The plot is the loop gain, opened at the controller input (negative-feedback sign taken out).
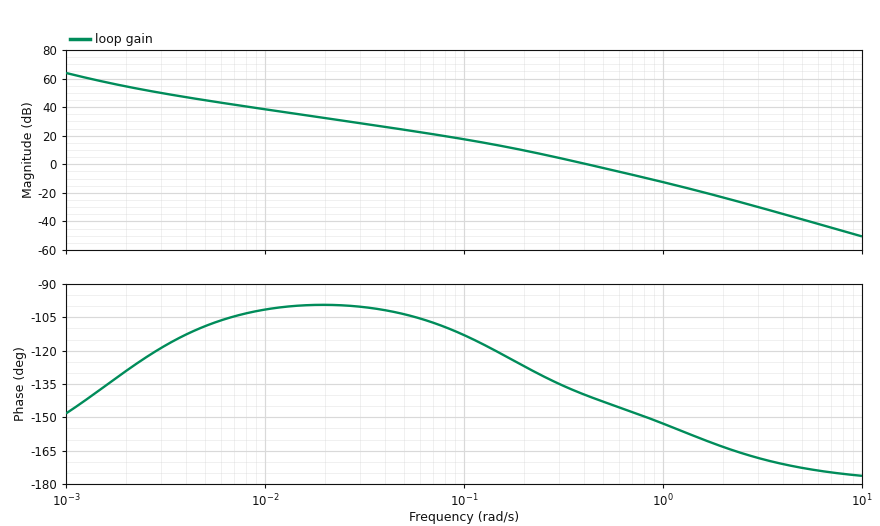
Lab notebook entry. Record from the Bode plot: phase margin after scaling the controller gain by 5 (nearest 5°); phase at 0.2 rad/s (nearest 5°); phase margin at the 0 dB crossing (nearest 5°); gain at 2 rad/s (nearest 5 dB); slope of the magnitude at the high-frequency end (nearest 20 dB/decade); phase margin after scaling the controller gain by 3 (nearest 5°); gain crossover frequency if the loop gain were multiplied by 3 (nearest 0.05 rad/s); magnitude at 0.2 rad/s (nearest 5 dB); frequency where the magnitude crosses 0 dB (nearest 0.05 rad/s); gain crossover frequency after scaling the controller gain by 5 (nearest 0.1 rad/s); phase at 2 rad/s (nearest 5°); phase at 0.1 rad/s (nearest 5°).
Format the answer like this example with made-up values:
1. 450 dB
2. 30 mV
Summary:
1. 25°
2. -125°
3. 40°
4. -25 dB
5. -40 dB/decade
6. 30°
7. 0.80 rad/s
8. 10 dB
9. 0.40 rad/s
10. 1.1 rad/s
11. -165°
12. -115°
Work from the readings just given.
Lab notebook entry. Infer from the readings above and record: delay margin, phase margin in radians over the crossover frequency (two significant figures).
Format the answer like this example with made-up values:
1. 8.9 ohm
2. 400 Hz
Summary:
1. 1.7 s
